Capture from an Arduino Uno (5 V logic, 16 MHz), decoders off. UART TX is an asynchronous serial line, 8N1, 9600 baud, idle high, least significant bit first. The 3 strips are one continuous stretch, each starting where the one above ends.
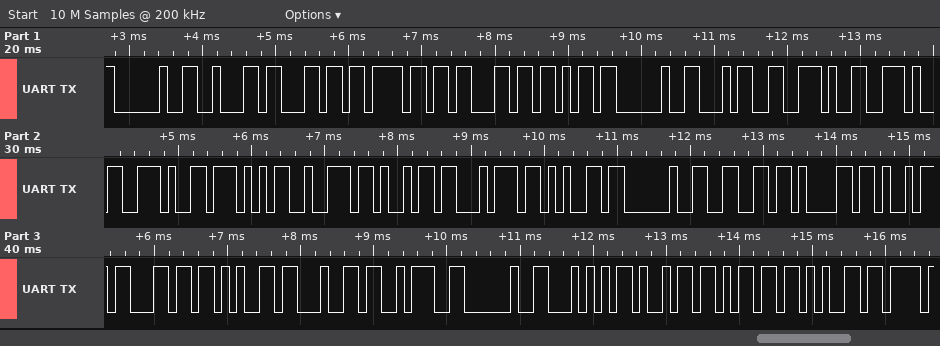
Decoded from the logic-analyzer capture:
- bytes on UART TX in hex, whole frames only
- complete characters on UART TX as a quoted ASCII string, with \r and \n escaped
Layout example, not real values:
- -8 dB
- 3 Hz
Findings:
- 20 62 6C 6F 63 6B 20 34 2E 2E 2E 57 72 69 74 65 20 66 61 69 6C 65 64 3A 20 54 69 6D 65
- " block 4...Write failed: Time"
